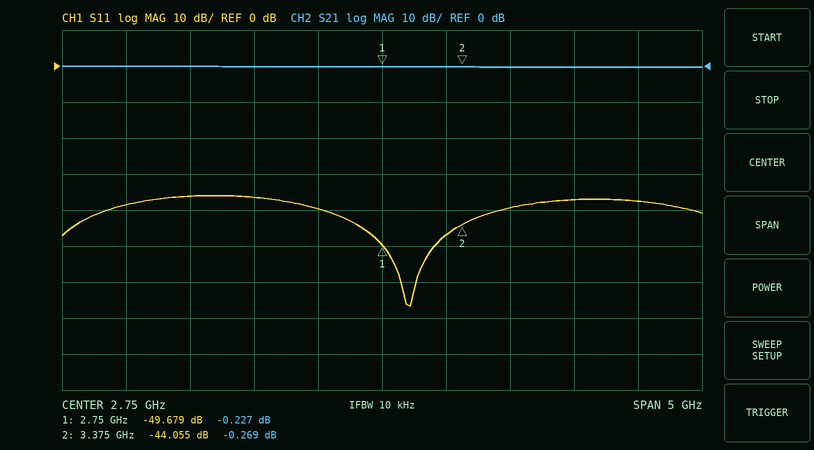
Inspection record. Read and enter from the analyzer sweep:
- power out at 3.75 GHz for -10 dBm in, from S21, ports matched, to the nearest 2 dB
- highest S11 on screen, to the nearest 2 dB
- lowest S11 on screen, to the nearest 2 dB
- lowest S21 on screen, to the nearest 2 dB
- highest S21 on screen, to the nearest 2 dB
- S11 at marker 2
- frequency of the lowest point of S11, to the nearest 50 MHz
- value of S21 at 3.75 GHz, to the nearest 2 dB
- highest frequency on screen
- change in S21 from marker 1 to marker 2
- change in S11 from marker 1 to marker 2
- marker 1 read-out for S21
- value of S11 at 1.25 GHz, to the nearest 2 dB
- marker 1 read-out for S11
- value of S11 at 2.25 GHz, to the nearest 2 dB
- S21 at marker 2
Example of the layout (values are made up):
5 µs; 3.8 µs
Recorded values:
-10 dBm; -36 dB; -66 dB; 0 dB; 0 dB; -44.055 dB; 2.95 GHz; 0 dB; 5.25 GHz; -0.042 dB; 5.624 dB; -0.227 dB; -36 dB; -49.679 dB; -40 dB; -0.269 dB
